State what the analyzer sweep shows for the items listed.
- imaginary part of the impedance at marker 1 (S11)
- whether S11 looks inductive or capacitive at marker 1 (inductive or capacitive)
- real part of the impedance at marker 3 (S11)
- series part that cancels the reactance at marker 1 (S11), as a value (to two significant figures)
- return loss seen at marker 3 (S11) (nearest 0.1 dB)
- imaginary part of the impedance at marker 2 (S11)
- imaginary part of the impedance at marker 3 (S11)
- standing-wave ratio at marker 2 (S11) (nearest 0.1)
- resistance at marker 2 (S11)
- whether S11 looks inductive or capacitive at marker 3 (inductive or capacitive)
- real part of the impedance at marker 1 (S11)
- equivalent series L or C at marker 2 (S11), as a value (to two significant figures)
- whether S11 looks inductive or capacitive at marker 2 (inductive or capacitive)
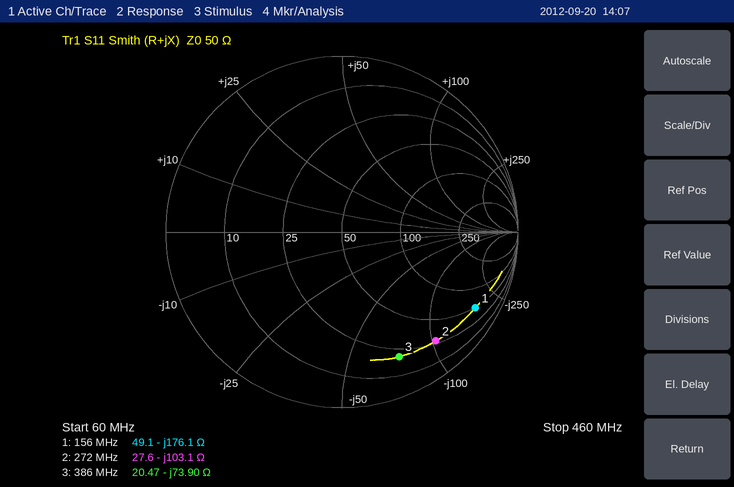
-176.1 Ω
capacitive
20.47 Ω
180 nH
2.2 dB
-103.1 Ω
-73.90 Ω
10.0
27.6 Ω
capacitive
49.1 Ω
5.7 pF
capacitive
